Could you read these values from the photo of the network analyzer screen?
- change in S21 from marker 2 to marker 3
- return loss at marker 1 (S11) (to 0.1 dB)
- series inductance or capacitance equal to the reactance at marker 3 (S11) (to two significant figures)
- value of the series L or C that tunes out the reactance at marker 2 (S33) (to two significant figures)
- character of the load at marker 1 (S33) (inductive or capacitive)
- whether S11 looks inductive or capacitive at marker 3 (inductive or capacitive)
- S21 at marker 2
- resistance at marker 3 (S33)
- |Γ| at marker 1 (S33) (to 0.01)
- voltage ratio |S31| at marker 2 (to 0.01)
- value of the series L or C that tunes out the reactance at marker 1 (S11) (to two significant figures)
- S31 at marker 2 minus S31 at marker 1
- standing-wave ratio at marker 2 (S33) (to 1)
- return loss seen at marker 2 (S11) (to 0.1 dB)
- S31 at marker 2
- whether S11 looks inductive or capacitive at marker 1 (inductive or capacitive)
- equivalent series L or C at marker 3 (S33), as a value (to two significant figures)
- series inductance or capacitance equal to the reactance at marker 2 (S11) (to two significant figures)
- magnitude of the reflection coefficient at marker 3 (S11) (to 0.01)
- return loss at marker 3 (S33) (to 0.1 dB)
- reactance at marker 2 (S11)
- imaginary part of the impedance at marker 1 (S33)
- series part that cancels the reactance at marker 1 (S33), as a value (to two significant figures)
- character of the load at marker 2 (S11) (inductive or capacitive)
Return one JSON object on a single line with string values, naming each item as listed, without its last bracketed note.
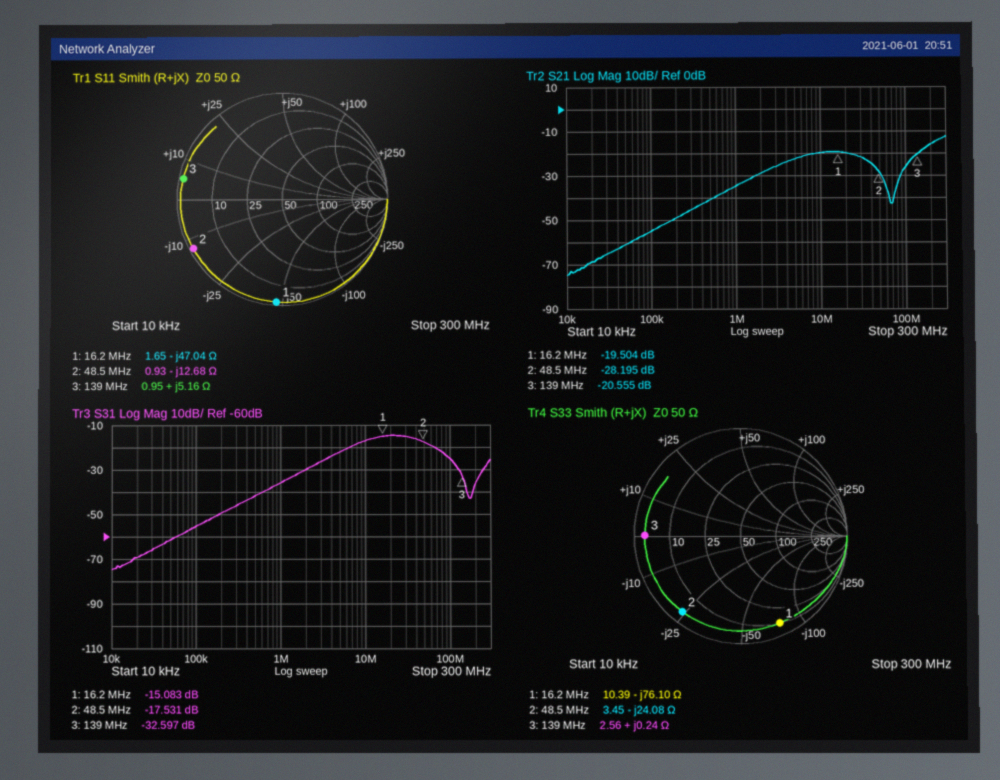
{"change in S21 from marker 2 to marker 3": "7.640 dB", "return loss at marker 1 (S11)": "0.3 dB", "series inductance or capacitance equal to the reactance at marker 3 (S11)": "5.9 nH", "value of the series L or C that tunes out the reactance at marker 2 (S33)": "79 nH", "character of the load at marker 1 (S33)": "capacitive", "whether S11 looks inductive or capacitive at marker 3": "inductive", "S21 at marker 2": "-28.195 dB", "resistance at marker 3": "2.56 Ω", "|Γ| at marker 1 (S33)": "0.88", "voltage ratio |S31| at marker 2": "0.13", "value of the series L or C that tunes out the reactance at marker 1 (S11)": "460 nH", "S31 at marker 2 minus S31 at marker 1": "-2.448 dB", "standing-wave ratio at marker 2 (S33)": "18", "return loss seen at marker 2 (S11)": "0.3 dB", "S31 at marker 2": "-17.531 dB", "whether S11 looks inductive or capacitive at marker 1": "capacitive", "equivalent series L or C at marker 3 (S33), as a value": "270 pH", "series inductance or capacitance equal to the reactance at marker 2 (S11)": "260 pF", "magnitude of the reflection coefficient at marker 3 (S11)": "0.96", "return loss at marker 3 (S33)": "0.9 dB", "reactance at marker 2": "-12.68 Ω", "imaginary part of the impedance at marker 1": "-76.10 Ω", "series part that cancels the reactance at marker 1 (S33), as a value": "750 nH", "character of the load at marker 2 (S11)": "capacitive"}
